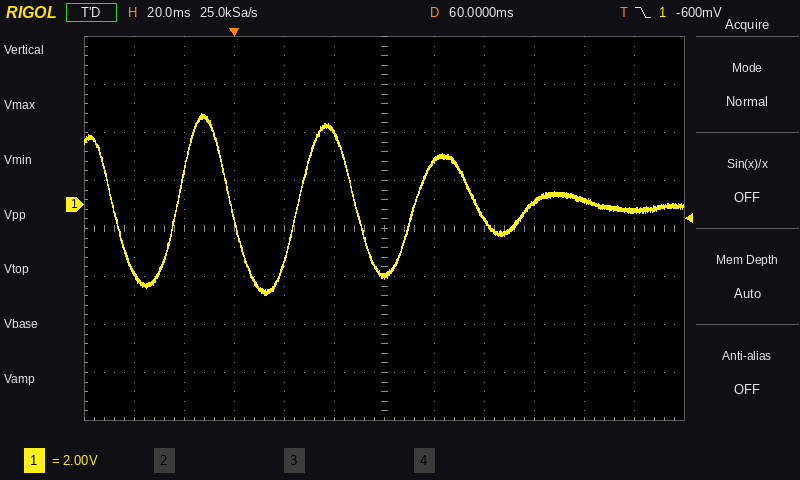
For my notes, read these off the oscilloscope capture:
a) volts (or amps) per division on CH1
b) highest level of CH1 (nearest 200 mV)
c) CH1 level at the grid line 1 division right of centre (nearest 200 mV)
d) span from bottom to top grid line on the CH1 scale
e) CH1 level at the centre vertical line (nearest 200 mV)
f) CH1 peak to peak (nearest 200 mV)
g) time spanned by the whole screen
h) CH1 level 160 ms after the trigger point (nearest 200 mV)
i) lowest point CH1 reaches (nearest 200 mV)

2 V
3.8 V
1.8 V
16 V
-3.0 V
7.6 V
240 ms
-200 mV
-3.8 V
